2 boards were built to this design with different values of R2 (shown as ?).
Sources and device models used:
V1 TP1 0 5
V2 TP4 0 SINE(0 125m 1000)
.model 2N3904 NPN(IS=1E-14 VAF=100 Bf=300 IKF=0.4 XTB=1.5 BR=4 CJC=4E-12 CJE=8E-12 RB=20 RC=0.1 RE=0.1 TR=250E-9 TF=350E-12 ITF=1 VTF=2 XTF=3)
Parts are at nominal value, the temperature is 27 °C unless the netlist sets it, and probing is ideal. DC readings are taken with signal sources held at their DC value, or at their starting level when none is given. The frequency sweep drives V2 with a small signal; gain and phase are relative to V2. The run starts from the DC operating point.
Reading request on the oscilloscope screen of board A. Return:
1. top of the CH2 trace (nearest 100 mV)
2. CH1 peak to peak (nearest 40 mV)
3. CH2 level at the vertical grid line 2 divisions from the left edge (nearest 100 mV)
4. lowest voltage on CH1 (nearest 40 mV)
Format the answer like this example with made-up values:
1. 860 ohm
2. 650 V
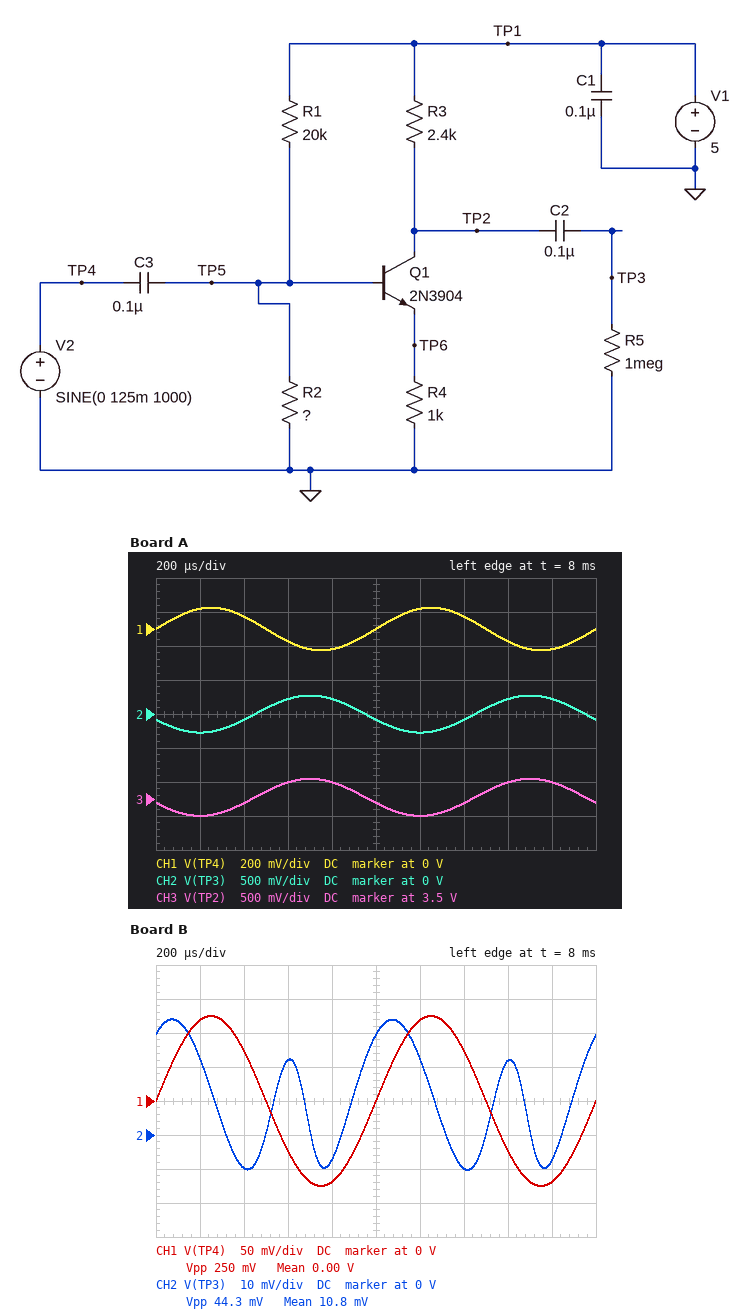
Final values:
1. 300 mV
2. 240 mV
3. -100 mV
4. -120 mV
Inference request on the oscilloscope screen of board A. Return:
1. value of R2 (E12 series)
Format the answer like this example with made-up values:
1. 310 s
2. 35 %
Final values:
1. 6.8 kΩ
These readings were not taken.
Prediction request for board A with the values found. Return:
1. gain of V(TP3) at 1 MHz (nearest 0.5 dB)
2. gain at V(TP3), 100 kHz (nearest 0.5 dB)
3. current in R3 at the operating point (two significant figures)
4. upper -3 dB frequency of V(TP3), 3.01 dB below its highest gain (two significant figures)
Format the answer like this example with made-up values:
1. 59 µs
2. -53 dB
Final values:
1. 7.0 dB
2. 7.0 dB
3. 610 µA
4. 38 MHz
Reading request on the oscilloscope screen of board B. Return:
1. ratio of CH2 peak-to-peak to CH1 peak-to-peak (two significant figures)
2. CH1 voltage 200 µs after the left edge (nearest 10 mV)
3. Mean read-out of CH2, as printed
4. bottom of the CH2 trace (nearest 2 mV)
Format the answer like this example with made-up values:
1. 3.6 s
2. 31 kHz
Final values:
1. 0.18
2. 120 mV
3. 10.8 mV
4. -10 mV
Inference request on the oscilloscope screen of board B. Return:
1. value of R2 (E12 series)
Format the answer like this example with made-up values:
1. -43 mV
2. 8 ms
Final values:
1. 27 kΩ
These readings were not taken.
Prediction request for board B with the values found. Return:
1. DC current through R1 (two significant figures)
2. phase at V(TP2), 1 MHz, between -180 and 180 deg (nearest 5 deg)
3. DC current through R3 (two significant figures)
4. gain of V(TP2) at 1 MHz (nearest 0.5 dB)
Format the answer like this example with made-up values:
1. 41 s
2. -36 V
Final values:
1. 140 µA
2. 5 deg
3. 1.4 mA
4. -0.5 dB
